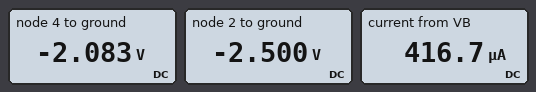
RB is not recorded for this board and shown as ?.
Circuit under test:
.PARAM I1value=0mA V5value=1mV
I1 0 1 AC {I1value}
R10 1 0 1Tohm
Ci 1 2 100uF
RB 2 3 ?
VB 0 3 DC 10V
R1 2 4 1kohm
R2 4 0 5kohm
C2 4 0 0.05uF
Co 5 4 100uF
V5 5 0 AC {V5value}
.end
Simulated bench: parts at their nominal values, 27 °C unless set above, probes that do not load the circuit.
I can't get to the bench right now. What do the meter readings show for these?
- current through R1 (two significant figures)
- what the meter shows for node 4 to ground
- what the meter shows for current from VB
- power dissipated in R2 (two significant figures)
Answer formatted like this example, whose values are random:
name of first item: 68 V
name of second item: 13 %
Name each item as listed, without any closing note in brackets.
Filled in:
current through R1: 420 µA
what the meter shows for node 4 to ground: -2.083 V
what the meter shows for current from VB: 416.7 µA
power dissipated in R2: 870 µW
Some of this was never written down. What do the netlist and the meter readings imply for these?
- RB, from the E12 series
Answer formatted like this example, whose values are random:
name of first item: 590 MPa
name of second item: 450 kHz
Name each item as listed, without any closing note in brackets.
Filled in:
RB, from the E12 series: 18 kΩ
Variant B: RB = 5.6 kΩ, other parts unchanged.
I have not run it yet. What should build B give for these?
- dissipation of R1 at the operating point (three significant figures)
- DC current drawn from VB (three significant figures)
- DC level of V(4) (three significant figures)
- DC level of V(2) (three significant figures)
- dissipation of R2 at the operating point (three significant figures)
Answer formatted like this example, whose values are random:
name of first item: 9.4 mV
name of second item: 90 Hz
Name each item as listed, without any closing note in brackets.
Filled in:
dissipation of R1 at the operating point: 743 µW
DC current drawn from VB: 862 µA
DC level of V(4): -4.31 V
DC level of V(2): -5.17 V
dissipation of R2 at the operating point: 3.72 mW
